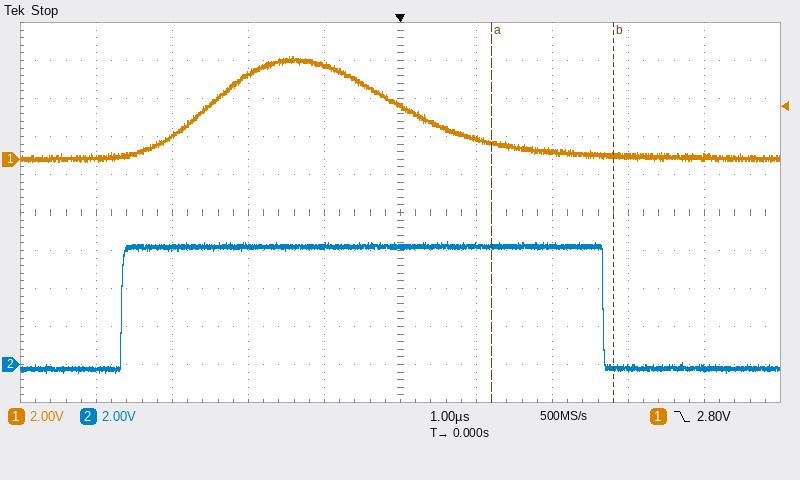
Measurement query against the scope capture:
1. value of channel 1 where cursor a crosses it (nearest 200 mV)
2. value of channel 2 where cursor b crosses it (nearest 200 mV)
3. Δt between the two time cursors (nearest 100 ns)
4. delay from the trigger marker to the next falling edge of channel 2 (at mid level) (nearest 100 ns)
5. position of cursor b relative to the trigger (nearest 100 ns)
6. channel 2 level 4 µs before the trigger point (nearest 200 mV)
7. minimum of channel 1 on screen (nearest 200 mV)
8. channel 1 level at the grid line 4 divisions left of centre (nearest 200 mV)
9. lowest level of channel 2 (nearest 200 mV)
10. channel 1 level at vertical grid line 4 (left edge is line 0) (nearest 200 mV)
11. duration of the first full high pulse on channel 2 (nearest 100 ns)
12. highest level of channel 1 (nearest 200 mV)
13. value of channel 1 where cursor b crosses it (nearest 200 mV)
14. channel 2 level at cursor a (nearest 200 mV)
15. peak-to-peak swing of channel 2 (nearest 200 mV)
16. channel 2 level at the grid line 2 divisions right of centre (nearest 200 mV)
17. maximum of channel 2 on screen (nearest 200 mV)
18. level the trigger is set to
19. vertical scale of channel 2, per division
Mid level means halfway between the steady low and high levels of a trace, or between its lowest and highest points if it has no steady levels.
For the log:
800 mV
-200 mV
1.6 µs
2.7 µs
+2.8 µs
-200 mV
-200 mV
0.0 V
-400 mV
5.0 V
6.3 µs
5.4 V
200 mV
6.2 V
6.8 V
6.2 V
6.4 V
2.80 V
2 V
